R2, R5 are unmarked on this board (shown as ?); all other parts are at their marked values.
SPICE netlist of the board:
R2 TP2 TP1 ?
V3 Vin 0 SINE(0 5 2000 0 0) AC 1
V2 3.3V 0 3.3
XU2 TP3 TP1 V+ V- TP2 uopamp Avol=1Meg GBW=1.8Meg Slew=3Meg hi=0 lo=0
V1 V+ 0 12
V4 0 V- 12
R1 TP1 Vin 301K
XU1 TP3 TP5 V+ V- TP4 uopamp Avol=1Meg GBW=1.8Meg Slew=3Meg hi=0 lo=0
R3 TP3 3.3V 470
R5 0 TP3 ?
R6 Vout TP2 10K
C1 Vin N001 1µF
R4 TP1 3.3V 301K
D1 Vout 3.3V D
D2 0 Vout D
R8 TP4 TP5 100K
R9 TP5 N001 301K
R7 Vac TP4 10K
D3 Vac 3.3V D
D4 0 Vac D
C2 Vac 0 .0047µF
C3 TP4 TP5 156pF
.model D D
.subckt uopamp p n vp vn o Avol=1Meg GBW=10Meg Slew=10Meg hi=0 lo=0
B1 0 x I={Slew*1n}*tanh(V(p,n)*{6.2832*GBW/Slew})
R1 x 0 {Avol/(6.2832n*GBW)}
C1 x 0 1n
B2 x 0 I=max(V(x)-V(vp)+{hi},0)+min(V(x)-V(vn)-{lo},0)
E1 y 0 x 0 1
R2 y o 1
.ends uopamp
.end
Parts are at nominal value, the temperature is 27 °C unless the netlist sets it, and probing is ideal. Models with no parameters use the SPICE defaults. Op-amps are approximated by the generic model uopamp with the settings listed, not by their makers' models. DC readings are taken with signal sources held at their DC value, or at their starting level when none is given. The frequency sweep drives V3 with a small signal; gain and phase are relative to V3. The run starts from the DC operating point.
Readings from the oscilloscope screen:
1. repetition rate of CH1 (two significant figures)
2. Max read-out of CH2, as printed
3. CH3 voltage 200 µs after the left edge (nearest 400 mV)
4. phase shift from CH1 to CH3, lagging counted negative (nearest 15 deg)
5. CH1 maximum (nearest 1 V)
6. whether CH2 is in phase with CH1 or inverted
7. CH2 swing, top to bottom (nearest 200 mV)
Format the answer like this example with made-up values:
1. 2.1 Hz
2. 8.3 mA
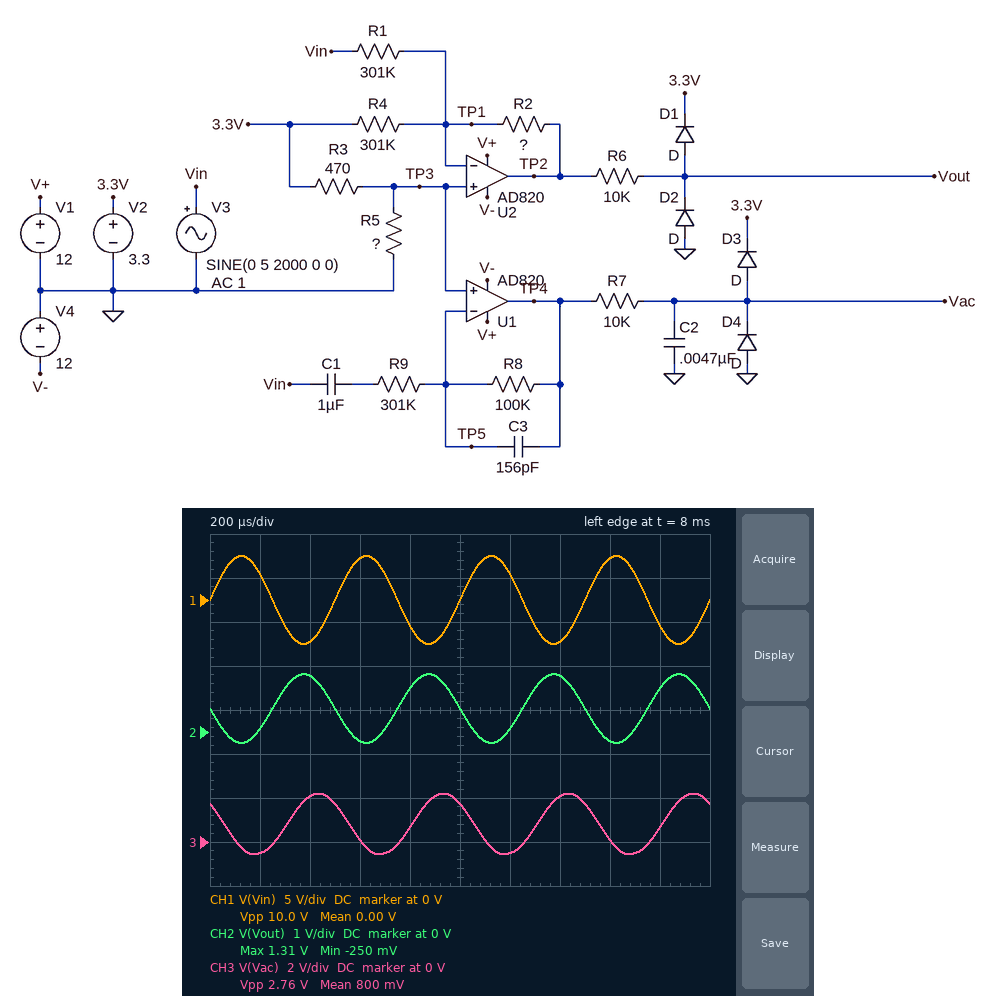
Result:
1. 2.0 kHz
2. 1.31 V
3. -400 mV
4. 135 deg
5. 5 V
6. inverted
7. 1.6 V
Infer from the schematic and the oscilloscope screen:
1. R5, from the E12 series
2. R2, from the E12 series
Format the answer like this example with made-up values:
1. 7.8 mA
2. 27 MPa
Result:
1. 150 Ω
2. 47 kΩ
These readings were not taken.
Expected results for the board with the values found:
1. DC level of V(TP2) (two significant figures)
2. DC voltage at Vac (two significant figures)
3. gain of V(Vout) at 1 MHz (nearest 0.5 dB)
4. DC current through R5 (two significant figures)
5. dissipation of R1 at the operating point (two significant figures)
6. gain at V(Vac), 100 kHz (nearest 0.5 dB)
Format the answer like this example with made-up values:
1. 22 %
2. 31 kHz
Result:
1. 530 mV
2. 800 mV
3. -18.0 dB
4. 5.3 mA
5. 2.1 µW
6. -59.0 dB
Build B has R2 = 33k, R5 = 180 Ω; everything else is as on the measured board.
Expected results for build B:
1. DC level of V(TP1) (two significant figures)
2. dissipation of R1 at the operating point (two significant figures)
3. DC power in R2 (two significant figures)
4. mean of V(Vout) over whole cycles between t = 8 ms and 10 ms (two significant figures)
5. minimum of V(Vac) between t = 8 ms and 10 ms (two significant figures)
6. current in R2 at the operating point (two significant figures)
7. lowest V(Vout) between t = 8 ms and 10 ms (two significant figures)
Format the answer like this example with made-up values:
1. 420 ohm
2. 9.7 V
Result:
1. 910 mV
2. 2.8 µW
3. 790 nW
4. 750 mV
5. -490 mV
6. 4.9 µA
7. 200 mV
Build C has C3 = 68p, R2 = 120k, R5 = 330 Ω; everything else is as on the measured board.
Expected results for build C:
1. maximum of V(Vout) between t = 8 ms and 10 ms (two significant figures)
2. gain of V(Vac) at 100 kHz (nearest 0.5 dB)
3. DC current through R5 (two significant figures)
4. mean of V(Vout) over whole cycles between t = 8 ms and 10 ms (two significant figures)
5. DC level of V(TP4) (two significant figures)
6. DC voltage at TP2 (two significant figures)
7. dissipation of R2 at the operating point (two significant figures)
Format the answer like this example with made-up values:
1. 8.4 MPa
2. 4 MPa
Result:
1. 3.1 V
2. -52.0 dB
3. 4.1 mA
4. 1.2 V
5. 1.4 V
6. 1.1 V
7. 440 nW
